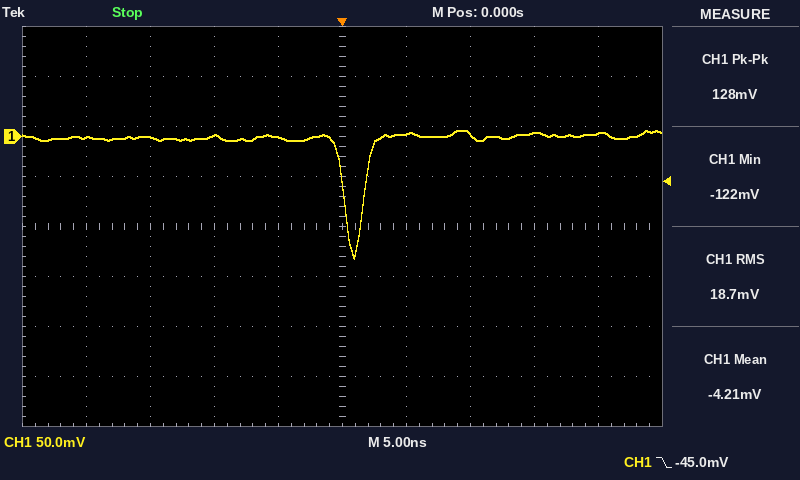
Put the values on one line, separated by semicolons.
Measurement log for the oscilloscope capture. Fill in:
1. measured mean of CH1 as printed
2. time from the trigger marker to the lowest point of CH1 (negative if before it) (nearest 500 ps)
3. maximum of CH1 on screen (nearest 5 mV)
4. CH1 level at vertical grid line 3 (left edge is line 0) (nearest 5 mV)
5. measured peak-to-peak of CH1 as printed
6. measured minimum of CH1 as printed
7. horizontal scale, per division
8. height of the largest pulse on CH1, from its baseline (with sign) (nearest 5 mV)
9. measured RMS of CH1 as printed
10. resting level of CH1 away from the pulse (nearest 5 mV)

-4.21 mV; +1.0 ns; 5 mV; 0 mV; 128 mV; -122 mV; 5 ns; -120 mV; 18.7 mV; 0 mV
